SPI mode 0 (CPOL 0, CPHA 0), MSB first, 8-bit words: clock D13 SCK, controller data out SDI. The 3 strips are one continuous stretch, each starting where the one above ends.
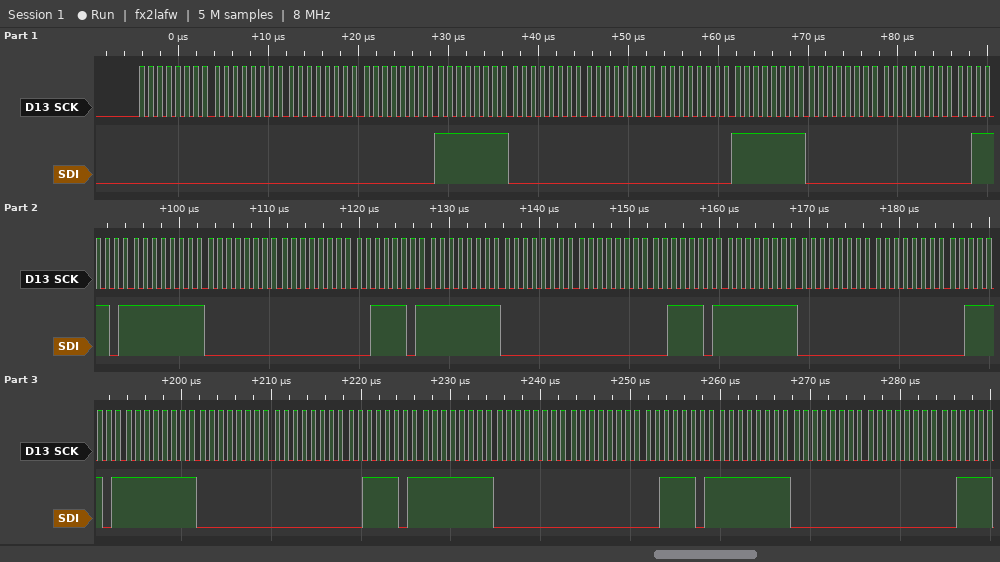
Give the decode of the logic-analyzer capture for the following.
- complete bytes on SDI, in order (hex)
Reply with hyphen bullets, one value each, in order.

- 0x00 0x00 0x00 0x00 0xFF 0x00 0x00 0x00 0xFF 0x00 0x00 0x3D 0xFF 0x00 0x00 0x3D 0xFF 0x00 0x00 0x3D 0xFF 0x00 0x00 0x3D 0xFF 0x00 0x00 0x3D 0xFF 0x00 0x00 0x3D 0xFF 0x00 0x00
